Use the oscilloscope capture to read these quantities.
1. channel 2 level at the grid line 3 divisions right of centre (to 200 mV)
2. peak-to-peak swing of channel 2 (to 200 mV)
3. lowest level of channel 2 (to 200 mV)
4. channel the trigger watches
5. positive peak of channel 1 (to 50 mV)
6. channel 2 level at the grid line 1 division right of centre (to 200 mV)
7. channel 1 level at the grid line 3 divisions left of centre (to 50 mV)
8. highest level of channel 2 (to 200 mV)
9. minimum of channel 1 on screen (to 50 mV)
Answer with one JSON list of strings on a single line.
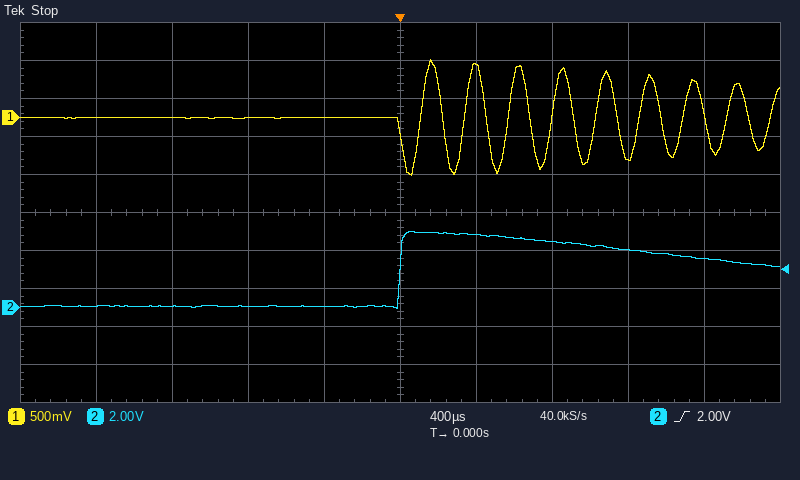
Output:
["3.0 V", "4.0 V", "0.0 V", "channel 2", "750 mV", "3.8 V", "0 mV", "4.0 V", "-750 mV"]
